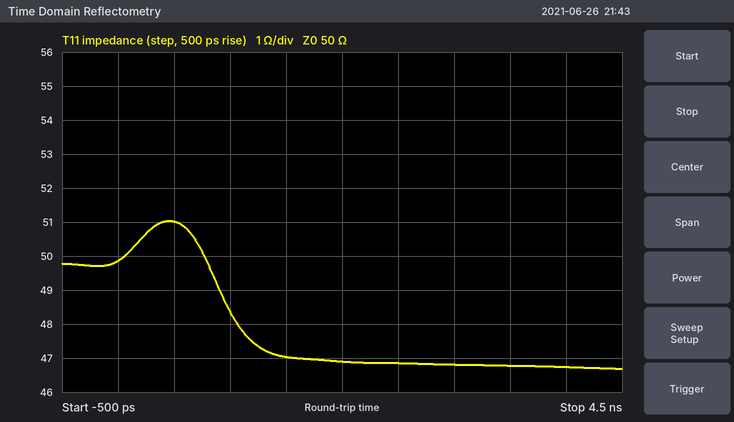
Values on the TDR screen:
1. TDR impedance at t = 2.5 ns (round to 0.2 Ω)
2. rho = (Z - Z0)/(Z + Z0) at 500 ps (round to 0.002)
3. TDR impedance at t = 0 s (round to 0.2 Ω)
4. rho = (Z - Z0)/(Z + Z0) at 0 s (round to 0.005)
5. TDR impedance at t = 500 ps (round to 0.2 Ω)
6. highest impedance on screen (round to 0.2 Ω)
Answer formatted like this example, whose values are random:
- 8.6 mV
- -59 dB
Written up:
- 46.8 Ω
- +0.010
- 49.8 Ω
- 0.000
- 51.0 Ω
- 51.0 Ω
